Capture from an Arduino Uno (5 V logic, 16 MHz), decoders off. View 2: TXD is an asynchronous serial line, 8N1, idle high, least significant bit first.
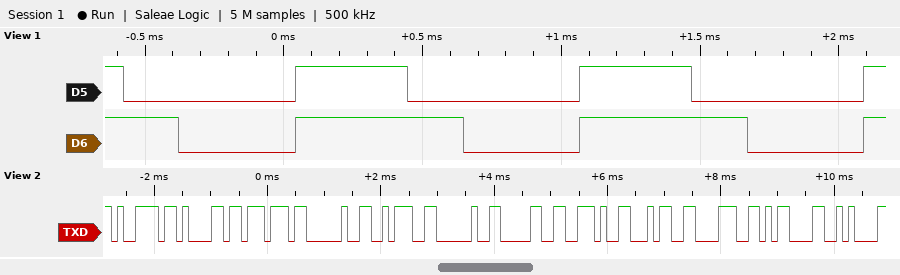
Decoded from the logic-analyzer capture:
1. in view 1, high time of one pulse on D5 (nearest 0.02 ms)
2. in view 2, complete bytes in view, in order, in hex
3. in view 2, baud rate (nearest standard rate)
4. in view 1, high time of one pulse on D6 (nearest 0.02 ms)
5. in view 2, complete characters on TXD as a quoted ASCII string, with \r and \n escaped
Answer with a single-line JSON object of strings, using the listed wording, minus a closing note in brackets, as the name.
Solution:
{"in view 1, high time of one pulse on D5": "0.40 ms", "in view 2, complete bytes in view, in order, in hex": "79 61 77 20 3A 20 30 2E 34 38 0D 0A", "in view 2, baud rate": "9600 baud", "in view 1, high time of one pulse on D6": "0.60 ms", "in view 2, complete characters on TXD as a quoted ASCII string, with \\r and \\n escaped": "\"yaw : 0.48\\r\\n\""}
